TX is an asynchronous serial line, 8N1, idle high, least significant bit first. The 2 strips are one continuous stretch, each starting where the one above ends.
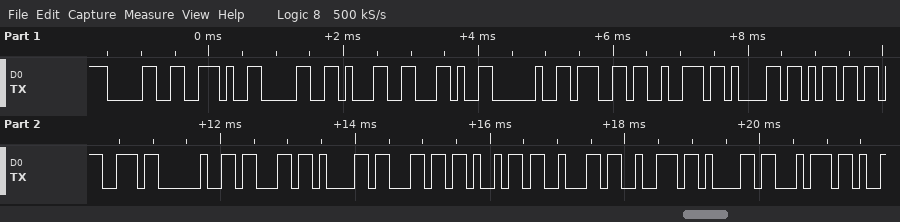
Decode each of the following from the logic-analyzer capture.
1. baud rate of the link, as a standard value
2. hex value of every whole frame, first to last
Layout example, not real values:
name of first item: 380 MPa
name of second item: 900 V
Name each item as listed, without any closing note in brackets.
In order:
baud rate of the link, as a standard value: 9600 baud
hex value of every whole frame, first to last: 0x30 0x2E 0x30 0x31 0x2C 0x20 0x67 0x72 0x61 0x6D 0x73 0x20 0x63 0x61 0x6C 0x69 0x62 0x72 0x61 0x74
